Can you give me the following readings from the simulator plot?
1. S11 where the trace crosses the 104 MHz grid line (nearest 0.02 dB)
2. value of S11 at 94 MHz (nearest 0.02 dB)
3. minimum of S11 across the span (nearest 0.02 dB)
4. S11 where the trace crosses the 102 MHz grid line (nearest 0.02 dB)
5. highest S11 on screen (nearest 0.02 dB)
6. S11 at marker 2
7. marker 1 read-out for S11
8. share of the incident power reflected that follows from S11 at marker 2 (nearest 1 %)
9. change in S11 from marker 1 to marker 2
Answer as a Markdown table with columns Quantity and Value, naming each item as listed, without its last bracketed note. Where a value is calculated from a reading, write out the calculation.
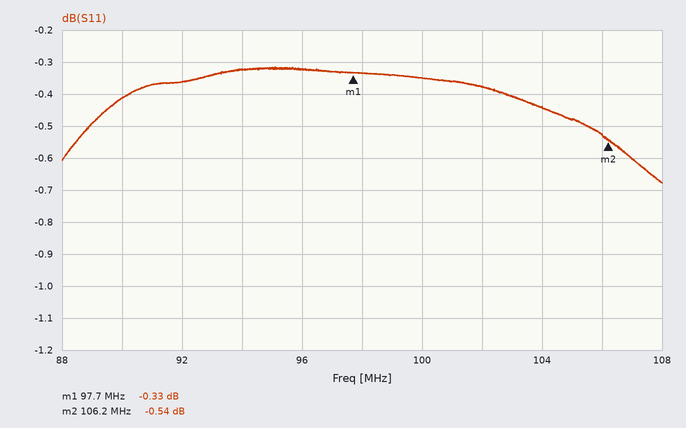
| Quantity | Value |
|---|---|
| S11 where the trace crosses the 104 MHz grid line | -0.44 dB |
| value of S11 at 94 MHz | -0.32 dB |
| minimum of S11 across the span | -0.68 dB |
| S11 where the trace crosses the 102 MHz grid line | -0.38 dB |
| highest S11 on screen | -0.32 dB |
| S11 at marker 2 | -0.54 dB |
| marker 1 read-out for S11 | -0.33 dB |
| share of the incident power reflected that follows from S11 at marker 2 | 10^(-0.54/10) ≈ 88 % |
| change in S11 from marker 1 to marker 2 | -0.54 − (-0.33) = -0.21 dB |
